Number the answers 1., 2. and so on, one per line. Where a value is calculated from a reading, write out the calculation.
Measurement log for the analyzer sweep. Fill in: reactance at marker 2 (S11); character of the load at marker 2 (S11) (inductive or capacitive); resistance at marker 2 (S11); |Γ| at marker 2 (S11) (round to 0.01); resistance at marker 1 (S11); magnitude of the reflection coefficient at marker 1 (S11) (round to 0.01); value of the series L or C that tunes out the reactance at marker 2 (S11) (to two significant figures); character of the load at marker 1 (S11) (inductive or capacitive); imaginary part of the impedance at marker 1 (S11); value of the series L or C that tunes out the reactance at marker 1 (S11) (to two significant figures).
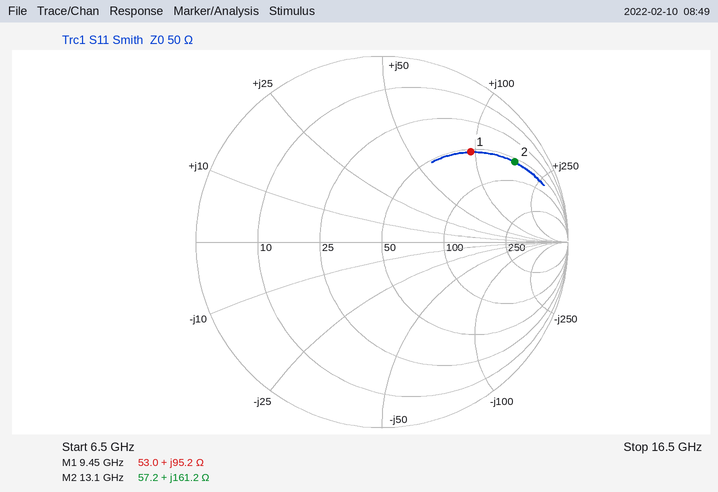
1. +161.2 Ω
2. inductive
3. 57.2 Ω
4. 0.83
5. 53.0 Ω
6. 0.68
7. C = 1/(2π × 13.1 GHz × 161.2 Ω) ≈ 75 fF
8. inductive
9. +95.2 Ω
10. C = 1/(2π × 9.45 GHz × 95.2 Ω) ≈ 177 fF, so 180 fF to two significant figures
